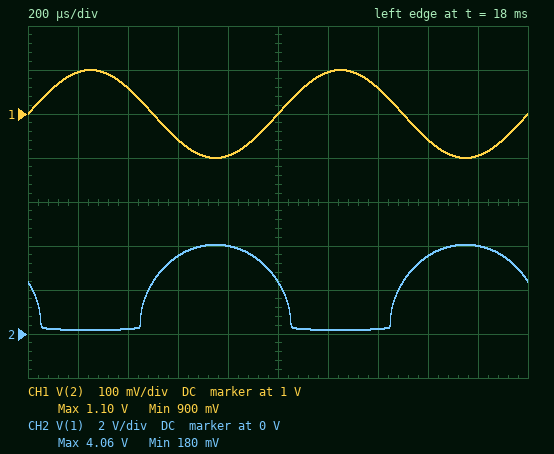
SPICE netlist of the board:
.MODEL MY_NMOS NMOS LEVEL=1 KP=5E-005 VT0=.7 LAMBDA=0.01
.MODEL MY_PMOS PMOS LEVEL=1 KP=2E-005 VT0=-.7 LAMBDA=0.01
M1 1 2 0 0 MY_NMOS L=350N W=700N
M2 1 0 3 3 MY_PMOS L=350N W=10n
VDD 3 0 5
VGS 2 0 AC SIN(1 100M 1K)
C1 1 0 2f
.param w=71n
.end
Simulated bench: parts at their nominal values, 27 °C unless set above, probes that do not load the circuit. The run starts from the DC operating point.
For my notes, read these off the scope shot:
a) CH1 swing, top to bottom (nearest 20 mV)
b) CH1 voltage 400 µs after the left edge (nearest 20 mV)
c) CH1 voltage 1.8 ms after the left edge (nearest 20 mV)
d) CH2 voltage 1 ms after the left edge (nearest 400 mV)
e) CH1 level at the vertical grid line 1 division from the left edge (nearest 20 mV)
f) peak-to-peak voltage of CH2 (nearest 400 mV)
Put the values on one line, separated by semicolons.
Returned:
200 mV; 1.06 V; 900 mV; 2.4 V; 1.10 V; 4.0 V
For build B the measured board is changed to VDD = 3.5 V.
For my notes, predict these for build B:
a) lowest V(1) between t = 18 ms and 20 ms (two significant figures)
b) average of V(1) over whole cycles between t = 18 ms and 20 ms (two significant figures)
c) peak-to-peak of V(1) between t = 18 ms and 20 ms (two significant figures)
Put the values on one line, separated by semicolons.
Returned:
63 mV; 320 mV; 1.6 V
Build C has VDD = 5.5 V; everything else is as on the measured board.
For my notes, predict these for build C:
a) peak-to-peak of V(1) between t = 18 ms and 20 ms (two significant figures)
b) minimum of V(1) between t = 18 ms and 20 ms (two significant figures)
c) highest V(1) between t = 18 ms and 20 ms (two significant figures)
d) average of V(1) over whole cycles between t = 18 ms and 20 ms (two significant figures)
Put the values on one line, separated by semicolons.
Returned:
4.4 V; 250 mV; 4.7 V; 2.8 V
